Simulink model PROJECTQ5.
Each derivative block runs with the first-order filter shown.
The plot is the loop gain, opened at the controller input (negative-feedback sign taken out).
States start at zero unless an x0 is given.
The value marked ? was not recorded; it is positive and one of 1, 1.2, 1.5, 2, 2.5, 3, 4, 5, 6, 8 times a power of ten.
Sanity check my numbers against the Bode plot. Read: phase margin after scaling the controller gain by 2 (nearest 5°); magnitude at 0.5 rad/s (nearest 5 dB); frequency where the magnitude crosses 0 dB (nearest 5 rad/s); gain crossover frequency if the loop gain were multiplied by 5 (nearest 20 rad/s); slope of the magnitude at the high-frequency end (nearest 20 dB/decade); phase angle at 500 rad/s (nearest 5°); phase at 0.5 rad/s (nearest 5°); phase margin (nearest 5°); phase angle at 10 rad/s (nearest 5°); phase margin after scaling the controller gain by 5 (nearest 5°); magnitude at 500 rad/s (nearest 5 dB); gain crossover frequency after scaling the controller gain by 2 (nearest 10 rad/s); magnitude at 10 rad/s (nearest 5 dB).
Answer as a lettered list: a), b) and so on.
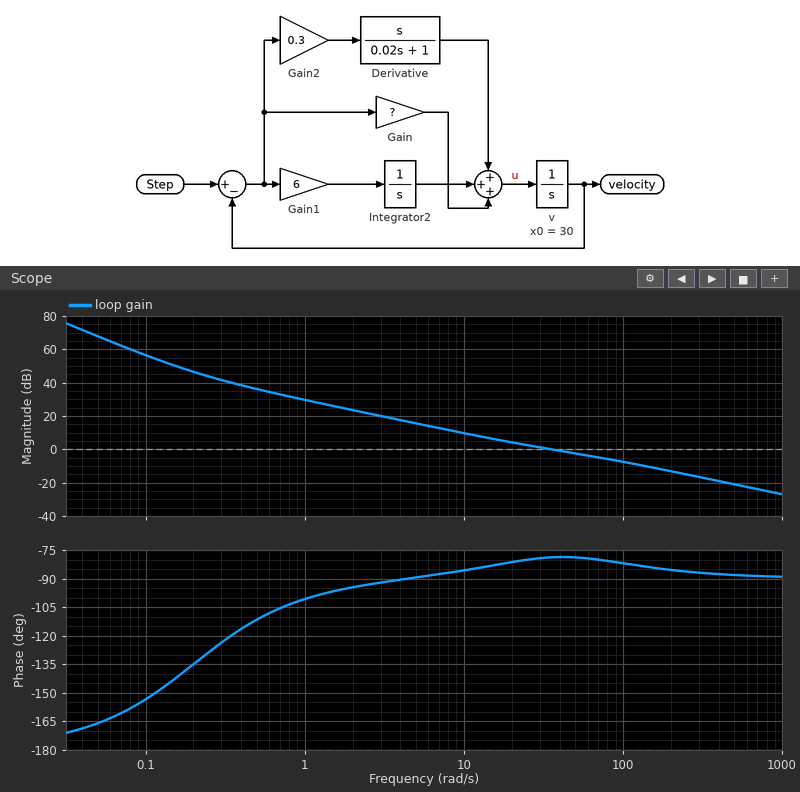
a) 100°
b) 35 dB
c) 35 rad/s
d) 220 rad/s
e) -20 dB/decade
f) -90°
g) -110°
h) 100°
i) -85°
j) 95°
k) -20 dB
l) 80 rad/s
m) 10 dB
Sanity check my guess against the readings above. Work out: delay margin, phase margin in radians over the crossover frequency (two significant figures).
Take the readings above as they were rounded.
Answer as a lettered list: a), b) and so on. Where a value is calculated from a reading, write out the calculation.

a) 100 × π / 180 / 35 = 0.050 s
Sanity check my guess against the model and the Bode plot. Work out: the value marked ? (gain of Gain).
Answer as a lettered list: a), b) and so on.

a) 30
